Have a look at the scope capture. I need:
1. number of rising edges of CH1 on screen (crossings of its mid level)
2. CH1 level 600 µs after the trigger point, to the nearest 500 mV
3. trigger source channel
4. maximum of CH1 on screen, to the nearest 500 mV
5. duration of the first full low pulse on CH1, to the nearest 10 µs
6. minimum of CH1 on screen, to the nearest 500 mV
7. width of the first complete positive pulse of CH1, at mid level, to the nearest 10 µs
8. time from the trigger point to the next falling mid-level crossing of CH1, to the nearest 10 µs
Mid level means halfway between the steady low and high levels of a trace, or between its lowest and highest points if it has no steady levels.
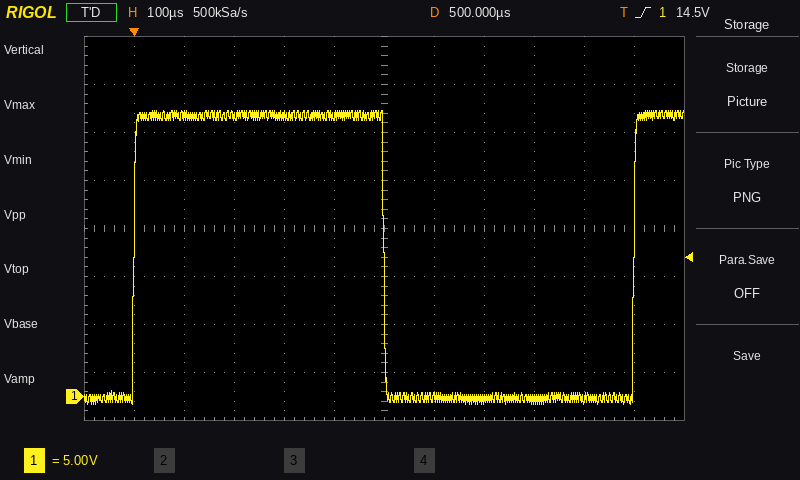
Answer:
2
0.0 V
CH1
30.0 V
500 µs
-1.0 V
500 µs
500 µs
